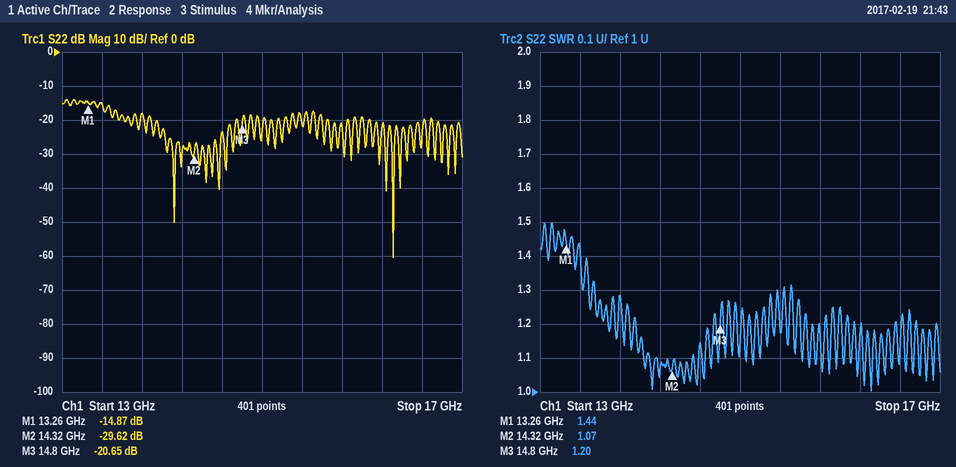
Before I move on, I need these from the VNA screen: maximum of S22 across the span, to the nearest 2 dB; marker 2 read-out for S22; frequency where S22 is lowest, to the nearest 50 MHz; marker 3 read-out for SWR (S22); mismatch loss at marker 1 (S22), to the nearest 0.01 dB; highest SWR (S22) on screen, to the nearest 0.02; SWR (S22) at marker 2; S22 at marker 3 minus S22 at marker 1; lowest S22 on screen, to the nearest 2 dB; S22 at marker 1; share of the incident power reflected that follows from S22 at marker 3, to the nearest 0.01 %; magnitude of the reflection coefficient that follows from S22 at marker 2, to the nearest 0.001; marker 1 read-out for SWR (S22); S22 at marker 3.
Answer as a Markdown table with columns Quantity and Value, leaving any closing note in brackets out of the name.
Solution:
| Quantity | Value |
|---|---|
| maximum of S22 across the span, to the nearest 2 dB | -14 dB |
| marker 2 read-out for S22 | -29.62 dB |
| frequency where S22 is lowest, to the nearest 50 MHz | 16.30 GHz |
| marker 3 read-out for SWR | 1.20 |
| mismatch loss at marker 1 (S22), to the nearest 0.01 dB | 0.14 dB |
| highest SWR (S22) on screen, to the nearest 0.02 | 1.50 |
| SWR (S22) at marker 2 | 1.07 |
| S22 at marker 3 minus S22 at marker 1 | -5.78 dB |
| lowest S22 on screen, to the nearest 2 dB | -60 dB |
| S22 at marker 1 | -14.87 dB |
| share of the incident power reflected that follows from S22 at marker 3, to the nearest 0.01 % | 0.86 % |
| magnitude of the reflection coefficient that follows from S22 at marker 2, to the nearest 0.001 | 0.033 |
| marker 1 read-out for SWR | 1.44 |
| S22 at marker 3 | -20.65 dB |
